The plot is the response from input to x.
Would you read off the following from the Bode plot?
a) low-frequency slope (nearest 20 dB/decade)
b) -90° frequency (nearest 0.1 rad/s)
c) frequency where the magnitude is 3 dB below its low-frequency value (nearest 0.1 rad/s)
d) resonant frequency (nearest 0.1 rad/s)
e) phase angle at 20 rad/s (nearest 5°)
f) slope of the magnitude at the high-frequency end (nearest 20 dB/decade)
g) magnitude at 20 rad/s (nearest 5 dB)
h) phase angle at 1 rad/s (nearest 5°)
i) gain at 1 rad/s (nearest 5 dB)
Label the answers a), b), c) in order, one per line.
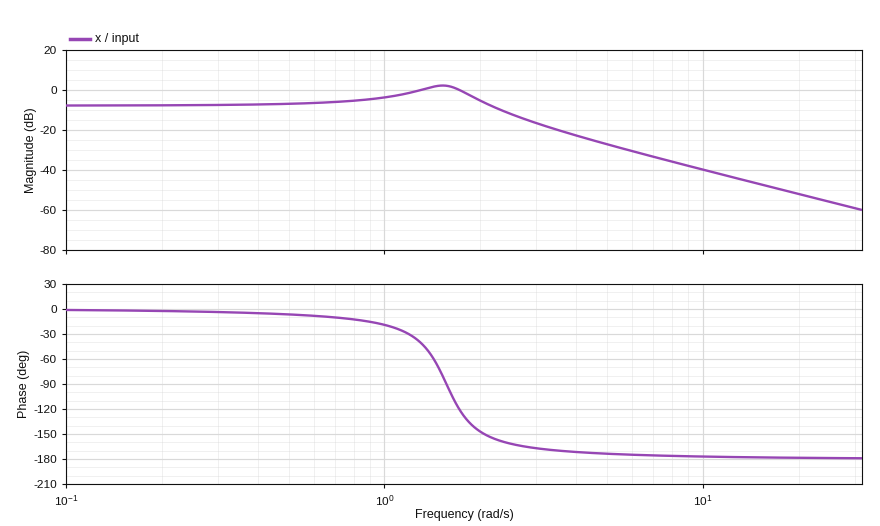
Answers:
a) 0 dB/decade
b) 1.6 rad/s
c) 2.4 rad/s
d) 1.5 rad/s
e) -180°
f) -40 dB/decade
g) -50 dB
h) -20°
i) -5 dB
